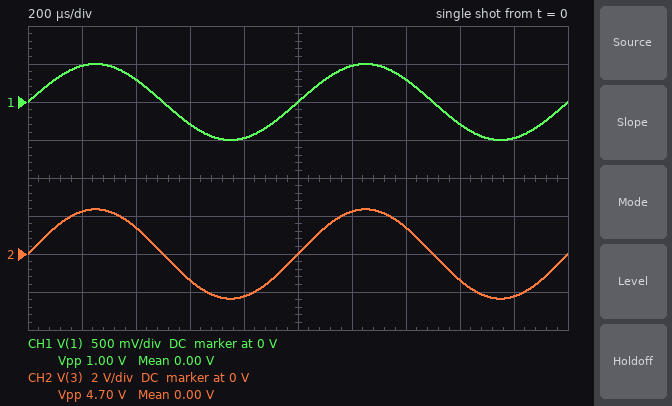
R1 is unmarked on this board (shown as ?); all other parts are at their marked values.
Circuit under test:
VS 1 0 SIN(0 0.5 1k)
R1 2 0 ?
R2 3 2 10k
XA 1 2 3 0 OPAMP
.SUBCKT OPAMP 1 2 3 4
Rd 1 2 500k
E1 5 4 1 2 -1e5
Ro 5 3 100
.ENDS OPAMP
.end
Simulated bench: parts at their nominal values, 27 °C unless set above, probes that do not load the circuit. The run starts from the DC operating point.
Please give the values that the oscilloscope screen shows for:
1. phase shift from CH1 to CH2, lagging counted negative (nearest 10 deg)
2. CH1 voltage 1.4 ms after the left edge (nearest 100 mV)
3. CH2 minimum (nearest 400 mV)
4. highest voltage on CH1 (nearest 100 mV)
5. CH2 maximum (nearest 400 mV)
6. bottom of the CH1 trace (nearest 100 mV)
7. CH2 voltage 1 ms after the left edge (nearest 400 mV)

0 deg
300 mV
-2.4 V
500 mV
2.4 V
-500 mV
0 V
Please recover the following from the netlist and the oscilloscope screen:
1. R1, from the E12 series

2.7 kΩ
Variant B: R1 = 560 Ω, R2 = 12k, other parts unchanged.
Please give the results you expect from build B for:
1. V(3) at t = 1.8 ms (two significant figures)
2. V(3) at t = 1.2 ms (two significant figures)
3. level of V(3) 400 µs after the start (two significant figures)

-11 V
11 V
6.6 V
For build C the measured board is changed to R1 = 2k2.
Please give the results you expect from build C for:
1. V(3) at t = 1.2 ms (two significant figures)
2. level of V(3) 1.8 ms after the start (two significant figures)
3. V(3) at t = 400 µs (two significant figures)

2.6 V
-2.6 V
1.6 V
